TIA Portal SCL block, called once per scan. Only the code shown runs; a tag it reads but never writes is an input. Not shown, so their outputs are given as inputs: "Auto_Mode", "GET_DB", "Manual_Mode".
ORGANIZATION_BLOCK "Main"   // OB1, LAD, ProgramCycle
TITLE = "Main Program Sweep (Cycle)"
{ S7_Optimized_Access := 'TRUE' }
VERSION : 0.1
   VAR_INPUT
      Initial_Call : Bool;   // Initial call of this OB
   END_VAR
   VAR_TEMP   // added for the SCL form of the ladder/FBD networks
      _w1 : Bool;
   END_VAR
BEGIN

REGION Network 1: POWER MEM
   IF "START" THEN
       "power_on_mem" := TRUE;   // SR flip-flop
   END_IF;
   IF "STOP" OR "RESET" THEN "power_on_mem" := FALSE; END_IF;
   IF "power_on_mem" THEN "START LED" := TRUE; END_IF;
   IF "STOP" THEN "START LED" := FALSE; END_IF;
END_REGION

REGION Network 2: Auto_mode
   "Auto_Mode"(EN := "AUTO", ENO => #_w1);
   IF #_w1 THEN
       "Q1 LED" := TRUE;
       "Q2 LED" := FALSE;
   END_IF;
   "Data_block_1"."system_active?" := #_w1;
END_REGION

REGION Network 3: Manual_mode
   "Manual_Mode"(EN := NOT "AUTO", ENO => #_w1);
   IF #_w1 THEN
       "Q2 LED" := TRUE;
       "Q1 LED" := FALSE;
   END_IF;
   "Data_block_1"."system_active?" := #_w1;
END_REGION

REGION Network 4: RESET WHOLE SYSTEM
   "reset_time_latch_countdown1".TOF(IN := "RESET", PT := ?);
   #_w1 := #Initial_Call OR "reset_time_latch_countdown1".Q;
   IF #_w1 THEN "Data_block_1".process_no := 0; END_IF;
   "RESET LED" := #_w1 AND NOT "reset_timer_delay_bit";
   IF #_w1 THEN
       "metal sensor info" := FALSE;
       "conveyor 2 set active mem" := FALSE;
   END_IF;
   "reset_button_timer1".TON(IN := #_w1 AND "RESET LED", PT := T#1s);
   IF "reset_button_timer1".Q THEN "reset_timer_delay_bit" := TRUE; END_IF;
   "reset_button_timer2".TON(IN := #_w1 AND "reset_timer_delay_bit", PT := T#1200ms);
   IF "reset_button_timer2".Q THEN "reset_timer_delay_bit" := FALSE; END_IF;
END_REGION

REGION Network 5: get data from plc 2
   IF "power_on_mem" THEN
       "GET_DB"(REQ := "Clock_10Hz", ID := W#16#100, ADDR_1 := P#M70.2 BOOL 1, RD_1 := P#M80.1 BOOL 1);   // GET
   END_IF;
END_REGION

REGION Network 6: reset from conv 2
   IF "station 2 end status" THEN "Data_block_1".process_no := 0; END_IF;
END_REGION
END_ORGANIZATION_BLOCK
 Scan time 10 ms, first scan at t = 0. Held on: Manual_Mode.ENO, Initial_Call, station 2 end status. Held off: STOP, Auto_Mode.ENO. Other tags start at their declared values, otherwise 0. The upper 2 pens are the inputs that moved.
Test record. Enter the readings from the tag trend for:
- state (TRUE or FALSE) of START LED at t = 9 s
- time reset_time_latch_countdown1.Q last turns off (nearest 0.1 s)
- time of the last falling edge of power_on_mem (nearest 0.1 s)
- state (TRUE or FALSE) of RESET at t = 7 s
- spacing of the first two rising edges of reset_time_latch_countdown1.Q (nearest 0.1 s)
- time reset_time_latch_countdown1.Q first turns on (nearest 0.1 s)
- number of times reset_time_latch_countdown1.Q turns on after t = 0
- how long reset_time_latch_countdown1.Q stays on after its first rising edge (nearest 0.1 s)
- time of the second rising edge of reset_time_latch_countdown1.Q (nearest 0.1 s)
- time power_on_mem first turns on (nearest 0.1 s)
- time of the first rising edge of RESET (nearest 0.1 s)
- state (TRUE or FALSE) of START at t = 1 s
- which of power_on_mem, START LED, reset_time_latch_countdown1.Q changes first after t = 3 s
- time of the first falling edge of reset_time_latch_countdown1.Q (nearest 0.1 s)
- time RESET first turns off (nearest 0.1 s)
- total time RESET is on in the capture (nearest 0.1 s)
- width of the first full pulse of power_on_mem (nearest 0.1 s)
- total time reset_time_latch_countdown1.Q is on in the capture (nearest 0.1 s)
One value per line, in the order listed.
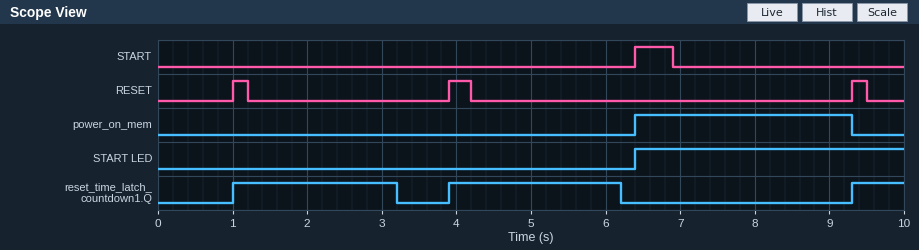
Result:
TRUE
6.2 s
9.3 s
FALSE
2.9 s
1.0 s
3
2.2 s
3.9 s
6.4 s
1.0 s
FALSE
reset_time_latch_countdown1.Q
3.2 s
1.2 s
0.7 s
2.9 s
5.2 s
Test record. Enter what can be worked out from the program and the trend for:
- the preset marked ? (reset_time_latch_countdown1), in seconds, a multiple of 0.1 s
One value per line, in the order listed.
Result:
2.0 s
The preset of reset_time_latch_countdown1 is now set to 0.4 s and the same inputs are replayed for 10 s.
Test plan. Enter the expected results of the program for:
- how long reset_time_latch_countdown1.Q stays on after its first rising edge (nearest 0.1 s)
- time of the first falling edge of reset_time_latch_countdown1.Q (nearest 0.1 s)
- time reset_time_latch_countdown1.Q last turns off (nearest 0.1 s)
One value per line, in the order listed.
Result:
0.6 s
1.6 s
9.9 s
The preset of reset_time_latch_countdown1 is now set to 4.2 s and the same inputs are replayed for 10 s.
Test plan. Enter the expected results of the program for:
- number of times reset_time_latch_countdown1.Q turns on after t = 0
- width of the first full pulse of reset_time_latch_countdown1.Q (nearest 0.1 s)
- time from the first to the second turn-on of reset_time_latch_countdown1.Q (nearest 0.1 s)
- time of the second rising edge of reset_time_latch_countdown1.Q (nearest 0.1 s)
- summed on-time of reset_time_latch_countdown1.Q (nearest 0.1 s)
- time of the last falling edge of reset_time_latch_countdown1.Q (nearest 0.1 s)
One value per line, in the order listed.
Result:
2
7.4 s
8.3 s
9.3 s
8.1 s
8.4 s
